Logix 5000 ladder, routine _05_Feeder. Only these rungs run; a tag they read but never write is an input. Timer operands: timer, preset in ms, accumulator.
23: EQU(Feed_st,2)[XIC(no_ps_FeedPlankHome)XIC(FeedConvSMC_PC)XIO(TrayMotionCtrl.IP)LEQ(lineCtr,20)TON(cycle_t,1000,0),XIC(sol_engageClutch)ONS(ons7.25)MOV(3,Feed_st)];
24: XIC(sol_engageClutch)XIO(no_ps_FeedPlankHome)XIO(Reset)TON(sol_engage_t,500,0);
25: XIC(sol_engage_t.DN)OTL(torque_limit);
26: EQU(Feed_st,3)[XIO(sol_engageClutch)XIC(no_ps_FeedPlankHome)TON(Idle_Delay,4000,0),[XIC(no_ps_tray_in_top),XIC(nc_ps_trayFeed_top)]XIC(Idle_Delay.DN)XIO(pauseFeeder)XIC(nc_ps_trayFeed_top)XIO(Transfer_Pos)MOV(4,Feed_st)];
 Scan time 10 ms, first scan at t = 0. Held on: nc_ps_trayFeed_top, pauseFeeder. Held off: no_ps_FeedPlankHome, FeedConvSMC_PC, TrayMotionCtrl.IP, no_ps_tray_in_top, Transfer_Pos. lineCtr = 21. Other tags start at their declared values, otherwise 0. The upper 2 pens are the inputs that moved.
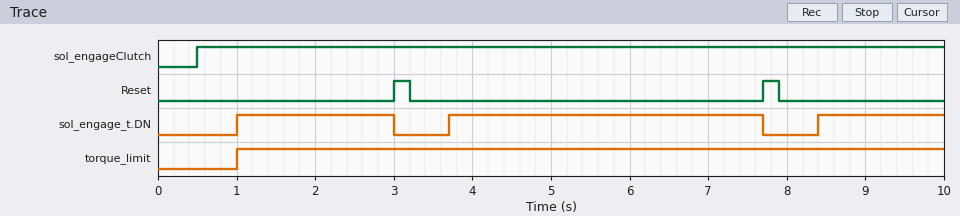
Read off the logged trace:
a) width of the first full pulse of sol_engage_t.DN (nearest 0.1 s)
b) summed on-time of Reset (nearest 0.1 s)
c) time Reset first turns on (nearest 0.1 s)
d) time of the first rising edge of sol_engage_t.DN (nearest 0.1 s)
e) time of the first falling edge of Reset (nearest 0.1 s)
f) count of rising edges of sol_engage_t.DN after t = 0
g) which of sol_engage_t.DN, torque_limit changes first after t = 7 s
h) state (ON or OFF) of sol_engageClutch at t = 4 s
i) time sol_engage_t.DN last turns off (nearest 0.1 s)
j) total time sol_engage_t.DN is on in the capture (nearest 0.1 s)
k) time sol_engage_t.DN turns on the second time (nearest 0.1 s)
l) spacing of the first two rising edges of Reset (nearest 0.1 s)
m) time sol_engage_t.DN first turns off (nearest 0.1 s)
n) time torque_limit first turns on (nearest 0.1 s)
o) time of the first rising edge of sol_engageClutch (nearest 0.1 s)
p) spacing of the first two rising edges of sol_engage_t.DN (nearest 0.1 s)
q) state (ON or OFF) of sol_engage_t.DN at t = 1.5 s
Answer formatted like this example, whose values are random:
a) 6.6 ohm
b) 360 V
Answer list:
a) 2.0 s
b) 0.4 s
c) 3.0 s
d) 1.0 s
e) 3.2 s
f) 3
g) sol_engage_t.DN
h) ON
i) 7.7 s
j) 7.6 s
k) 3.7 s
l) 4.7 s
m) 3.0 s
n) 1.0 s
o) 0.5 s
p) 2.7 s
q) ON
